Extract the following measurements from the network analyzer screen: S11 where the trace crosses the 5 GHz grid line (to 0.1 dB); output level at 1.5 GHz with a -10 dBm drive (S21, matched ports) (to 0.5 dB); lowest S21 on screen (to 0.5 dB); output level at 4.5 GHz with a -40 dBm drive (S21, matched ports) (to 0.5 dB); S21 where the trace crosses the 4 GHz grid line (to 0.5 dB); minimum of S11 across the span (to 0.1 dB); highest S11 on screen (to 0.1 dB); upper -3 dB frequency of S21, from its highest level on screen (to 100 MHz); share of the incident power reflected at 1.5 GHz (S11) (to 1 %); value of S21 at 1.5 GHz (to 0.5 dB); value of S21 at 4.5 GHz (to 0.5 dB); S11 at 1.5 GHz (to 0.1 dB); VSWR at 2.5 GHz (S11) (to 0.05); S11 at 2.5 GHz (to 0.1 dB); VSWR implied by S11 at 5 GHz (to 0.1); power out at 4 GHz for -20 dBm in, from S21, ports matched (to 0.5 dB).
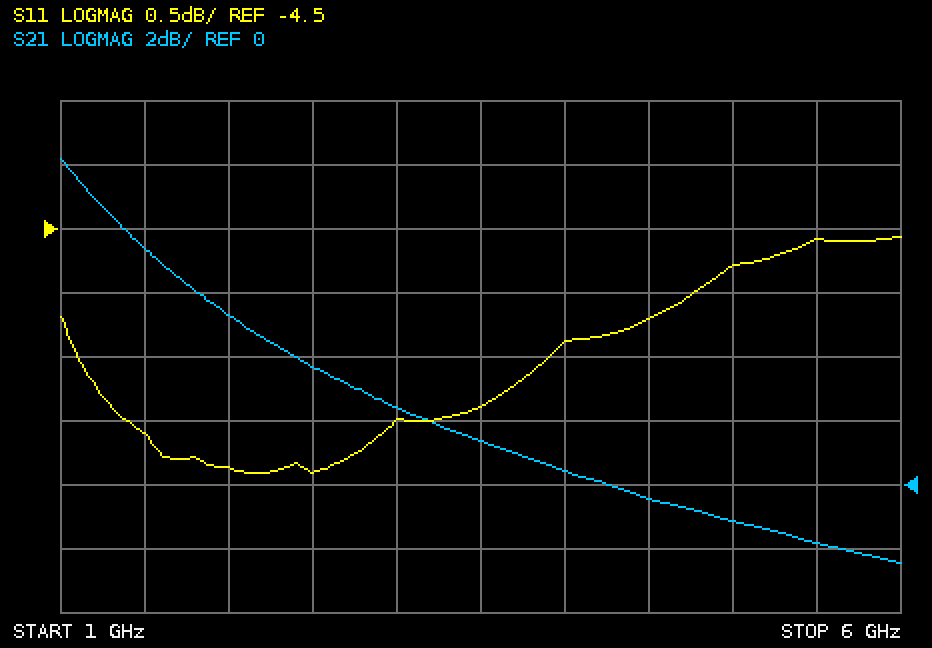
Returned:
-4.8 dB
-2.5 dBm
-2.5 dB
-40.5 dBm
0.5 dB
-6.4 dB
-4.6 dB
1.5 GHz
25 %
7.5 dB
-0.5 dB
-6.1 dB
2.85
-6.4 dB
3.7
-19.5 dBm
